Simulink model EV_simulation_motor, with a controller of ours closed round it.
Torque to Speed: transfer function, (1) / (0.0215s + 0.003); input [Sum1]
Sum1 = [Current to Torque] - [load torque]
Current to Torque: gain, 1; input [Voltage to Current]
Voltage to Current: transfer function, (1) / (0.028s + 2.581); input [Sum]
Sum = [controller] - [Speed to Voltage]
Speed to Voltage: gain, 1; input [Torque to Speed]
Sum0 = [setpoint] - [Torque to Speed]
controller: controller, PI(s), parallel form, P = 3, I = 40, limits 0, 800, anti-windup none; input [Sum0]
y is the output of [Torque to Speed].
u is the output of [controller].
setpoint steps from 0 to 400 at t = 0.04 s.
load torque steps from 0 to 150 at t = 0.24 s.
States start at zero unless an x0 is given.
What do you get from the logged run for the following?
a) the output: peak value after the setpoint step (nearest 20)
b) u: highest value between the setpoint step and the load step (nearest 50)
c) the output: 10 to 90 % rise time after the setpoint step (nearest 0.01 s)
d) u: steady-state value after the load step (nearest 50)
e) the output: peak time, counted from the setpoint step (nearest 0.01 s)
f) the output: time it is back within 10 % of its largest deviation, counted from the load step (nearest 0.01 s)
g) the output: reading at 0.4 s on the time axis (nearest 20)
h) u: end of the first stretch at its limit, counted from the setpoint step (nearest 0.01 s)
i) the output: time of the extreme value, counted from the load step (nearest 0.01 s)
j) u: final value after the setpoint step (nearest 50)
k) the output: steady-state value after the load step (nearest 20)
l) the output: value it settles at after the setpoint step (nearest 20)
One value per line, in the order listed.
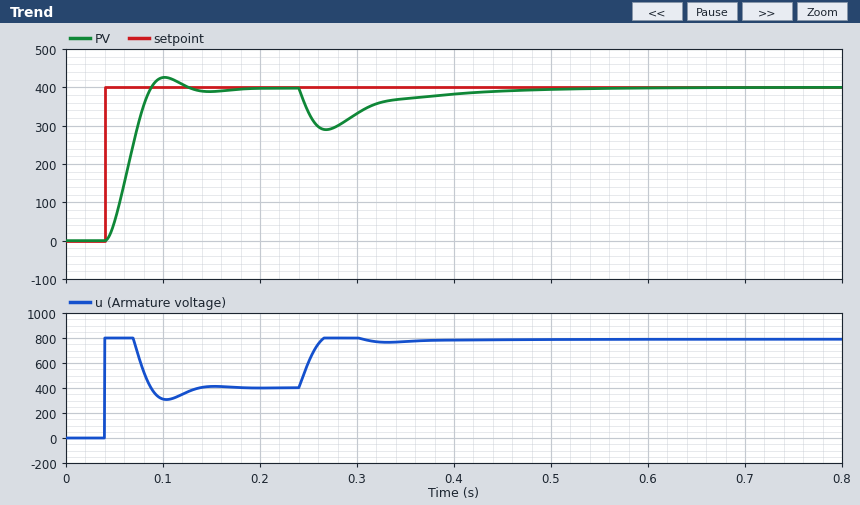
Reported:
420
800
0.03 s
800
0.06 s
0.20 s
380
0.03 s
0.03 s
400
400
400
